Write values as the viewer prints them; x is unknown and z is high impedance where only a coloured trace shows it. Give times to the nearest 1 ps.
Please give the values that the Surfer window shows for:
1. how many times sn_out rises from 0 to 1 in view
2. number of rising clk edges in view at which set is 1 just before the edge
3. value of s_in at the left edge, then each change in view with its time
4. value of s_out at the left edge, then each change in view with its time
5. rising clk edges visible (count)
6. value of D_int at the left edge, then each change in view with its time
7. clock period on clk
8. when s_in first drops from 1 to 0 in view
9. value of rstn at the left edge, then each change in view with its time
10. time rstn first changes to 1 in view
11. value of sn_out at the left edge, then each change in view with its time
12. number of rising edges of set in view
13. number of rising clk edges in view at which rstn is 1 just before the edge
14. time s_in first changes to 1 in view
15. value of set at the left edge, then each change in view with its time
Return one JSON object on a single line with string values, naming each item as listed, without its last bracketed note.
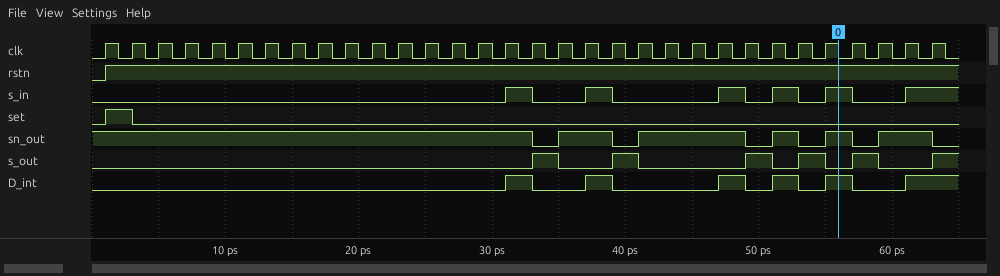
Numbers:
{"how many times sn_out rises from 0 to 1 in view": "5", "number of rising clk edges in view at which set is 1 just before the edge": "1", "value of s_in at the left edge, then each change in view with its time": "0, 1 at 31 ps, 0 at 33 ps, 1 at 37 ps, 0 at 39 ps, 1 at 47 ps, 0 at 49 ps, 1 at 51 ps, 0 at 53 ps, 1 at 55 ps, 0 at 57 ps, 1 at 61 ps", "value of s_out at the left edge, then each change in view with its time": "0, 1 at 33 ps, 0 at 35 ps, 1 at 39 ps, 0 at 41 ps, 1 at 49 ps, 0 at 51 ps, 1 at 53 ps, 0 at 55 ps, 1 at 57 ps, 0 at 59 ps, 1 at 63 ps", "rising clk edges visible": "32", "value of D_int at the left edge, then each change in view with its time": "0, 1 at 31 ps, 0 at 33 ps, 1 at 37 ps, 0 at 39 ps, 1 at 47 ps, 0 at 49 ps, 1 at 51 ps, 0 at 53 ps, 1 at 55 ps, 0 at 57 ps, 1 at 61 ps", "clock period on clk": "2 ps", "when s_in first drops from 1 to 0 in view": "33 ps", "value of rstn at the left edge, then each change in view with its time": "0, 1 at 1 ps", "time rstn first changes to 1 in view": "1 ps", "value of sn_out at the left edge, then each change in view with its time": "1, 0 at 33 ps, 1 at 35 ps, 0 at 39 ps, 1 at 41 ps, 0 at 49 ps, 1 at 51 ps, 0 at 53 ps, 1 at 55 ps, 0 at 57 ps, 1 at 59 ps, 0 at 63 ps", "number of rising edges of set in view": "1", "number of rising clk edges in view at which rstn is 1 just before the edge": "31", "time s_in first changes to 1 in view": "31 ps", "value of set at the left edge, then each change in view with its time": "0, 1 at 1 ps, 0 at 3 ps"}
